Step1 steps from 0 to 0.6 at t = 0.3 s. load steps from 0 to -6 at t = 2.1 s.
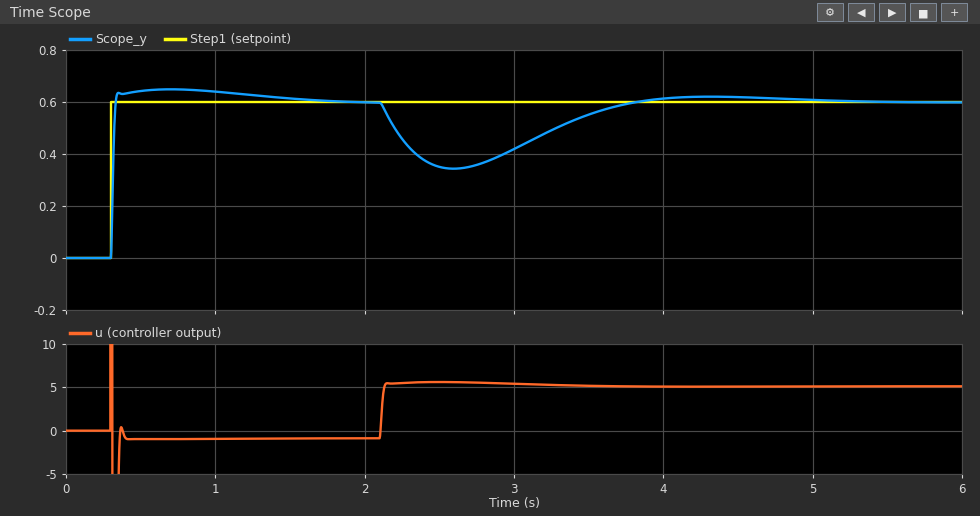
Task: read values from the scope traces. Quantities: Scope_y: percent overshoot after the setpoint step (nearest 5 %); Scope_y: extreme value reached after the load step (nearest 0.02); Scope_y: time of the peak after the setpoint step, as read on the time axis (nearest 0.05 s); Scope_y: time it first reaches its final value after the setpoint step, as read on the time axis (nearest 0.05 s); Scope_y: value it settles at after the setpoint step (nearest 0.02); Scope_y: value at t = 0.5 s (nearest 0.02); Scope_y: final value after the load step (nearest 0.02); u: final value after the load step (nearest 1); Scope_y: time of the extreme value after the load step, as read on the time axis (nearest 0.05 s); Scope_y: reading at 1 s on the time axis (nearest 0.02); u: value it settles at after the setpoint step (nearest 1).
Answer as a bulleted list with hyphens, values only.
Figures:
- 10 %
- 0.34
- 0.70 s
- 0.35 s
- 0.60
- 0.64
- 0.60
- 5
- 2.60 s
- 0.64
- -1
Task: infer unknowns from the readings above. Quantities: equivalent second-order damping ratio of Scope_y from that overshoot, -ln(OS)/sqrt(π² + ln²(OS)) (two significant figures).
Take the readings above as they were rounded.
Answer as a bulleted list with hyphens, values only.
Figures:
- 0.59
